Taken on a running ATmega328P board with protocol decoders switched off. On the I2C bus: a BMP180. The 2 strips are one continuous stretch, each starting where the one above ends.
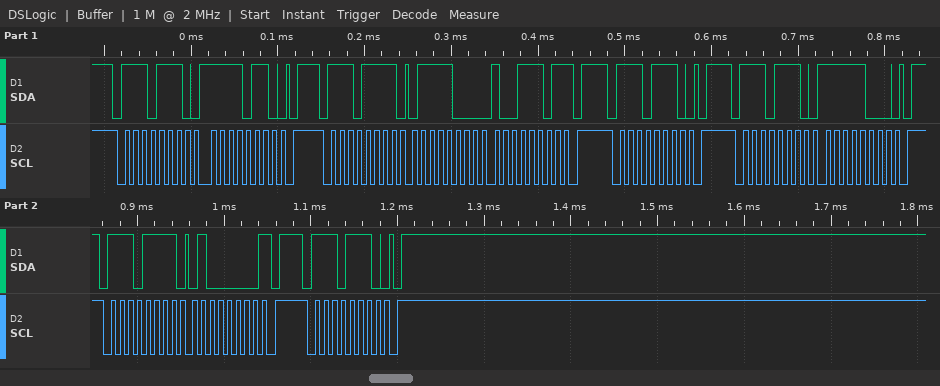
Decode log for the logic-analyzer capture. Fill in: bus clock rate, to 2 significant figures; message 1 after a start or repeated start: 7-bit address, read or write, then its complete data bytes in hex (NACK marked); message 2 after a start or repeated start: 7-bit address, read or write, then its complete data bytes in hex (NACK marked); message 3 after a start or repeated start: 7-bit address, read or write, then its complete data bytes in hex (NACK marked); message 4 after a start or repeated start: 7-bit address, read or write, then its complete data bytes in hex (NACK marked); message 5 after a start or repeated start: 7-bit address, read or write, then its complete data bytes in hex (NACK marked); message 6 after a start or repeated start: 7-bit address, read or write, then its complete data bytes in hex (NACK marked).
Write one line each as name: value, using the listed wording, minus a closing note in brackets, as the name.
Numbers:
bus clock rate, to 2 significant figures: 100 kHz
message 1 after a start or repeated start: 7-bit address, read or write, then its complete data bytes in hex: 0x77 write: F6
message 2 after a start or repeated start: 7-bit address, read or write, then its complete data bytes in hex: 0x77 read: 78 9D NACK
message 3 after a start or repeated start: 7-bit address, read or write, then its complete data bytes in hex: 0x77 write
message 4 after a start or repeated start: 7-bit address, read or write, then its complete data bytes in hex: 0x77 write: F8
message 5 after a start or repeated start: 7-bit address, read or write, then its complete data bytes in hex: 0x77 read: 40 NACK
message 6 after a start or repeated start: 7-bit address, read or write, then its complete data bytes in hex: 0x77 write
